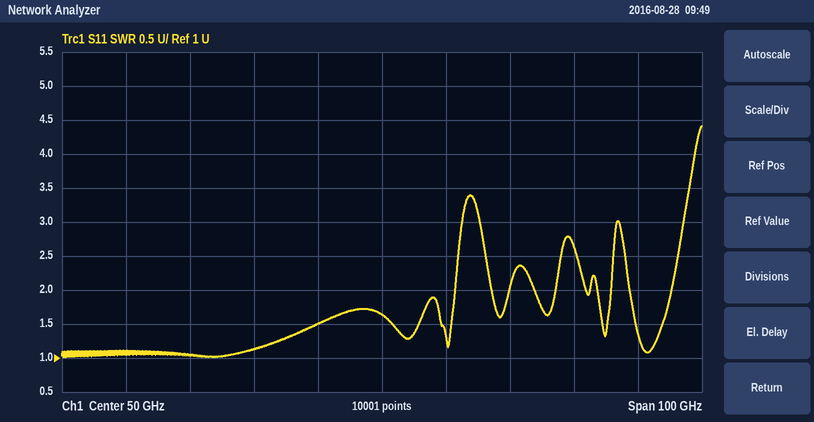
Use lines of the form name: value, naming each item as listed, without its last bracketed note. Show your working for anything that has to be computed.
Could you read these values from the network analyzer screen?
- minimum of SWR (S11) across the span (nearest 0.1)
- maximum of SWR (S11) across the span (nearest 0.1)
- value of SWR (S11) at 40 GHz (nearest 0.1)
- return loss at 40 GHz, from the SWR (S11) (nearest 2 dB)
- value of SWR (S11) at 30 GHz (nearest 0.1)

minimum of SWR (S11) across the span: 1.0
maximum of SWR (S11) across the span: 4.4
value of SWR (S11) at 40 GHz: 1.5
return loss at 40 GHz, from the SWR (S11): −20 log10((1.5 − 1)/(1.5 + 1)) ≈ 14 dB
value of SWR (S11) at 30 GHz: 1.1
